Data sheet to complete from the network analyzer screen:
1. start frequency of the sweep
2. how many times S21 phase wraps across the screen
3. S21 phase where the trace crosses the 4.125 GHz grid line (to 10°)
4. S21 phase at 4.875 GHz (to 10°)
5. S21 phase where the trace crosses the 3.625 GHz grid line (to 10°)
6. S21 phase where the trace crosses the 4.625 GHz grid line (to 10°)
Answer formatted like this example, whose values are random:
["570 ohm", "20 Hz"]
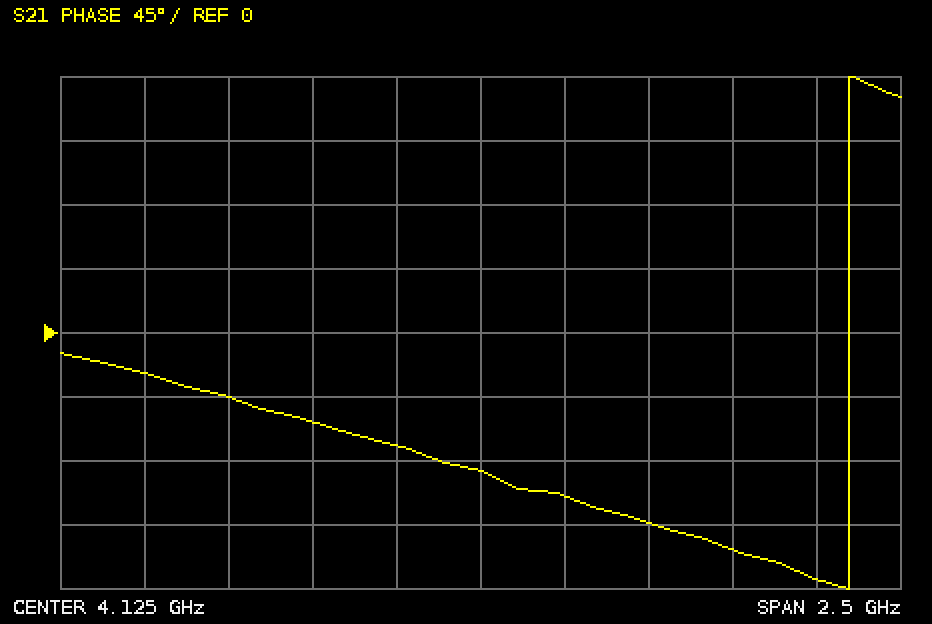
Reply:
["2.875 GHz", "1", "-100°", "-150°", "-60°", "-130°"]
